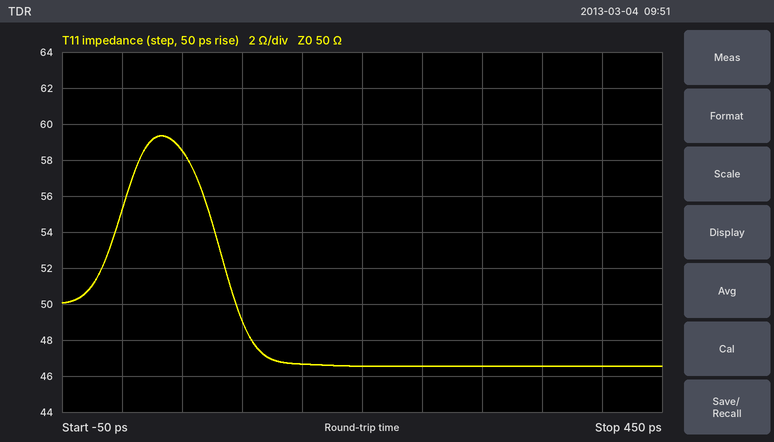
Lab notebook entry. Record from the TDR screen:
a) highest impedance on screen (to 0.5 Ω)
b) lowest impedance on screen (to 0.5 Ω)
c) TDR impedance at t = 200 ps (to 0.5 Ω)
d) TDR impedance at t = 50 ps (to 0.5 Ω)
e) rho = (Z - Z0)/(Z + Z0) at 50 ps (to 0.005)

59.5 Ω
46.5 Ω
46.5 Ω
58.5 Ω
+0.080
